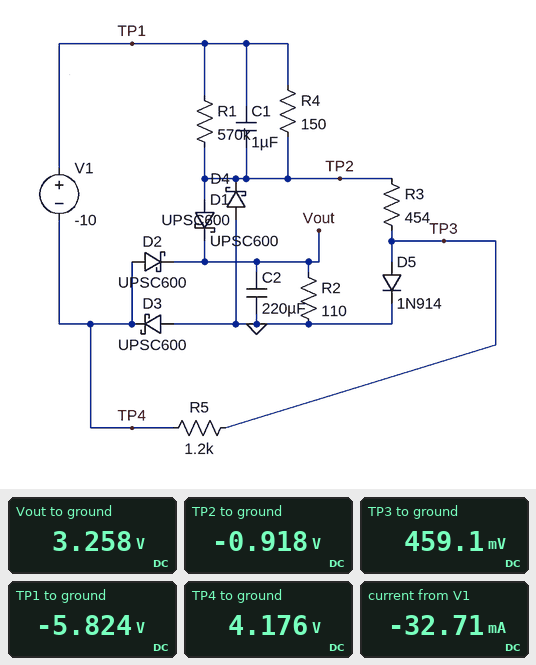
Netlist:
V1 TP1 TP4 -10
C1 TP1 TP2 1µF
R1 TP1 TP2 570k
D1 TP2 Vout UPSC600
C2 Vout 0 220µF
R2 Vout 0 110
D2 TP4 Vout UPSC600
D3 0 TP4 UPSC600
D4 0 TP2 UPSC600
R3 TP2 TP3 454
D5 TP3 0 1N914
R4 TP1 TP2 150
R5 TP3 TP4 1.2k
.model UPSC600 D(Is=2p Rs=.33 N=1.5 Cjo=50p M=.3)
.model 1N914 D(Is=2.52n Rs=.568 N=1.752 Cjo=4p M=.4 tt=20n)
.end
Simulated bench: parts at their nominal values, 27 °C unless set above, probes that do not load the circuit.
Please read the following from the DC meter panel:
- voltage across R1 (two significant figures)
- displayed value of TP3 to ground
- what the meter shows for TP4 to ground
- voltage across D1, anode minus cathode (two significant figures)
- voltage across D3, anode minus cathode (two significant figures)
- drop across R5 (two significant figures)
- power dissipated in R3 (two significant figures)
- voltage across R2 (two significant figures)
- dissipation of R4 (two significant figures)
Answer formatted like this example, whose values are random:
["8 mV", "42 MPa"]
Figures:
["4.9 V", "459.1 mV", "4.176 V", "-4.2 V", "-4.2 V", "3.7 V", "4.2 mW", "3.3 V", "160 mW"]
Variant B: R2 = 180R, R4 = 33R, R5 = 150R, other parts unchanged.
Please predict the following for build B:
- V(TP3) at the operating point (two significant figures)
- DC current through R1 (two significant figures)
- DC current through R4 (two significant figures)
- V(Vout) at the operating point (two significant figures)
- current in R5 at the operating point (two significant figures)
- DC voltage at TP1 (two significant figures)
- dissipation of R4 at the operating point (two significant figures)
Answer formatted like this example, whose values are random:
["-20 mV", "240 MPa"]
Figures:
["770 mV", "4.1 µA", "71 mA", "5.8 V", "39 mA", "-3.3 V", "170 mW"]
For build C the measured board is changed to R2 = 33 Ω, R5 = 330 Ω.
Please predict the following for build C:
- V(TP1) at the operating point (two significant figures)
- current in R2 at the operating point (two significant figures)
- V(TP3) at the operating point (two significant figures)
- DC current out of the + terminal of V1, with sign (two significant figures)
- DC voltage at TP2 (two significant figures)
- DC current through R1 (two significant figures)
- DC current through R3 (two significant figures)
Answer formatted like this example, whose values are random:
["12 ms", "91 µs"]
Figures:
["-7.7 V", "40 mA", "610 mV", "-45 mA", "-940 mV", "12 µA", "3.4 mA"]
